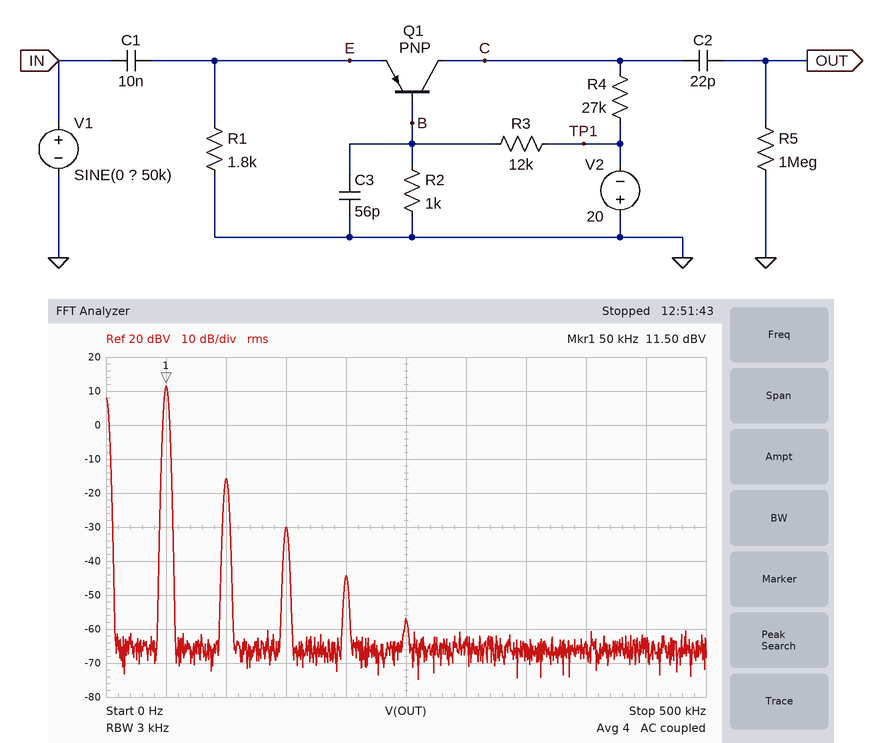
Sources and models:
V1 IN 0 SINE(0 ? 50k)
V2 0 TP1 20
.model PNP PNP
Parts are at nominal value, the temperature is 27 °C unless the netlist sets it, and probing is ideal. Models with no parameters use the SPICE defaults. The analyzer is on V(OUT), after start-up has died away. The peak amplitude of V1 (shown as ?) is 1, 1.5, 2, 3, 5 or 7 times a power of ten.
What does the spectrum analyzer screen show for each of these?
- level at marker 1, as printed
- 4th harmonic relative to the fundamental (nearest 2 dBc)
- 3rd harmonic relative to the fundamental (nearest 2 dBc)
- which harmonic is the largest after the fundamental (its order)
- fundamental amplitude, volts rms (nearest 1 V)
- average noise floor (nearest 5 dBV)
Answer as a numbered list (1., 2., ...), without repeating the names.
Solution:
1. 11.50 dBV
2. -56 dBc
3. -42 dBc
4. 2
5. 4 V
6. -65 dBV
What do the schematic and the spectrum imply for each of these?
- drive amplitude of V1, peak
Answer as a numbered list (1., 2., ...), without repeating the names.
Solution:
1. 70 mV
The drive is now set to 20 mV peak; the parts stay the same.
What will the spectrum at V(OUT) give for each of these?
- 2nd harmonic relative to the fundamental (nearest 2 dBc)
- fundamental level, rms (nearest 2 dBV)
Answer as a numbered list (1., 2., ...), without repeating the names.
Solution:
1. -38 dBc
2. 0 dBV
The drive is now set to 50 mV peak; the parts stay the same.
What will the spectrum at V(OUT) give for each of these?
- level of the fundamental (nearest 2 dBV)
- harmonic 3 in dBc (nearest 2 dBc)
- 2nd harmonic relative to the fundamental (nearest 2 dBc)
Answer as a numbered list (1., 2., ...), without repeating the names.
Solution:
1. 8 dBV
2. -48 dBc
3. -30 dBc
